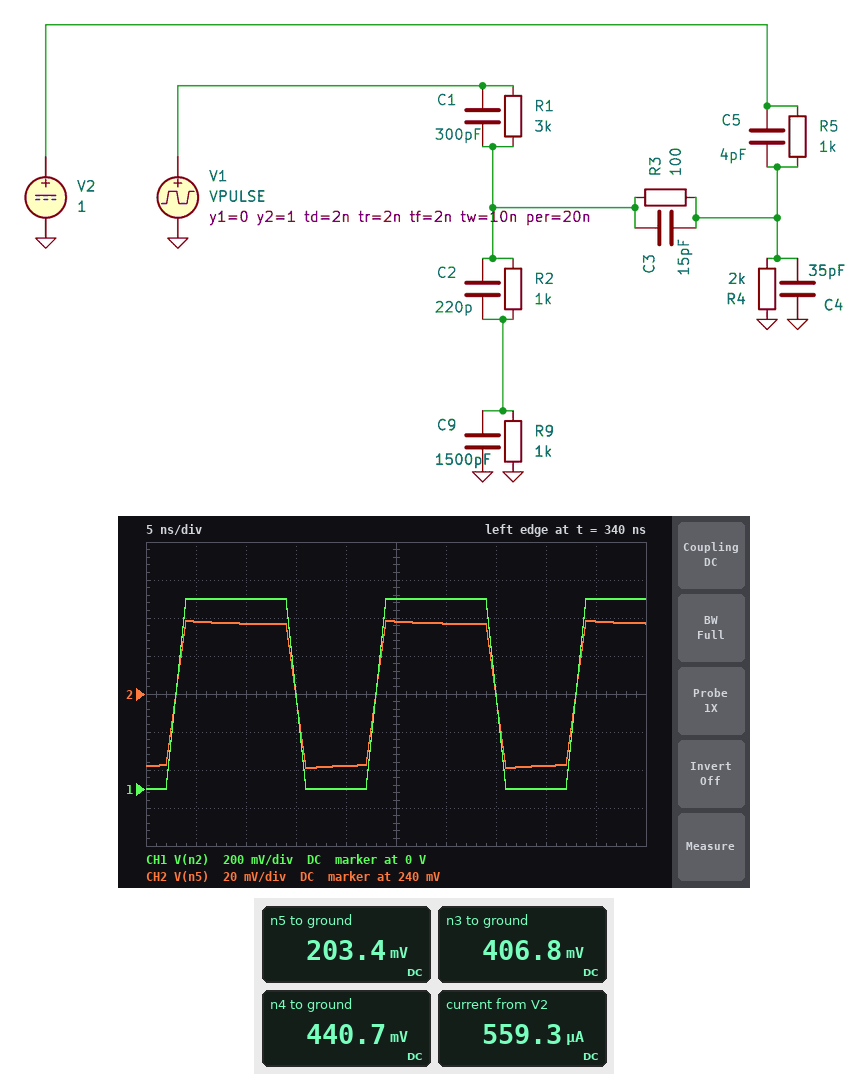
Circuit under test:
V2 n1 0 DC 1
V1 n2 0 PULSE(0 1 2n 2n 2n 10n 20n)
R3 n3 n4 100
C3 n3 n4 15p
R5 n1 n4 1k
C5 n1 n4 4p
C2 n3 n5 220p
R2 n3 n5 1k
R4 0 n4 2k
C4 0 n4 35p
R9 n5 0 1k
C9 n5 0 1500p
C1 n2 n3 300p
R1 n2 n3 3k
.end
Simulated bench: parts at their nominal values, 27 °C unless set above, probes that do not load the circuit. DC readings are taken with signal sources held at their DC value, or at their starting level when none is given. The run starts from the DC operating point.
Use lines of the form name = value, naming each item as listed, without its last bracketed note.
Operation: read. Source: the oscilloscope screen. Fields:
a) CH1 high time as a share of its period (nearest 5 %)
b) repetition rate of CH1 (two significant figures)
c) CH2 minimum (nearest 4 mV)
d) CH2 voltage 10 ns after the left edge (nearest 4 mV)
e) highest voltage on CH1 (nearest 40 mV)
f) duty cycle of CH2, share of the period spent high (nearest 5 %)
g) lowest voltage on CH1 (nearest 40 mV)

CH1 high time as a share of its period = 60 %
repetition rate of CH1 = 50 MHz
CH2 minimum = 200 mV
CH2 voltage 10 ns after the left edge = 276 mV
highest voltage on CH1 = 1.00 V
duty cycle of CH2, share of the period spent high = 60 %
lowest voltage on CH1 = 0 V
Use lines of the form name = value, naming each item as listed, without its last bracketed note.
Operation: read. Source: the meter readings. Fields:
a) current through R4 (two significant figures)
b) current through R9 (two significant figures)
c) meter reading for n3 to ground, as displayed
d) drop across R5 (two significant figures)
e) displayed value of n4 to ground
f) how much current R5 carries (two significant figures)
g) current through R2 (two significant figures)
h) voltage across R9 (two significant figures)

current through R4 = 220 µA
current through R9 = 200 µA
meter reading for n3 to ground, as displayed = 406.8 mV
drop across R5 = 560 mV
displayed value of n4 to ground = 440.7 mV
how much current R5 carries = 560 µA
current through R2 = 200 µA
voltage across R9 = 200 mV
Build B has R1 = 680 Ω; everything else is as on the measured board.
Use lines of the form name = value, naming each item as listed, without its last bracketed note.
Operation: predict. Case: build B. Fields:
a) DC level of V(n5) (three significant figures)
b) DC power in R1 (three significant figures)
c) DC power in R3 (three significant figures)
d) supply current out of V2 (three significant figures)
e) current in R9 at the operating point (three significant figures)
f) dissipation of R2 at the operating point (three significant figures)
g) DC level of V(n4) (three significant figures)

DC level of V(n5) = 133 mV
DC power in R1 = 104 µW
DC power in R3 = 27.4 µW
supply current out of V2 = 682 µA
current in R9 at the operating point = 133 µA
dissipation of R2 at the operating point = 17.6 µW
DC level of V(n4) = 318 mV
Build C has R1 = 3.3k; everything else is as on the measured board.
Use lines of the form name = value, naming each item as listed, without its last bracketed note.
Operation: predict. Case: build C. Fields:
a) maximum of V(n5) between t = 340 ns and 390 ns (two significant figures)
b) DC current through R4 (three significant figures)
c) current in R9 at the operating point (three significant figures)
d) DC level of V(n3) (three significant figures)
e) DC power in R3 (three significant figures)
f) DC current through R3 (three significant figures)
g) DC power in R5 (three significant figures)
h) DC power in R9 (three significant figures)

maximum of V(n5) between t = 340 ns and 390 ns = 280 mV
DC current through R4 = 223 µA
current in R9 at the operating point = 206 µA
DC level of V(n3) = 413 mV
DC power in R3 = 11.0 µW
DC current through R3 = 331 µA
DC power in R5 = 307 µW
DC power in R9 = 42.6 µW
